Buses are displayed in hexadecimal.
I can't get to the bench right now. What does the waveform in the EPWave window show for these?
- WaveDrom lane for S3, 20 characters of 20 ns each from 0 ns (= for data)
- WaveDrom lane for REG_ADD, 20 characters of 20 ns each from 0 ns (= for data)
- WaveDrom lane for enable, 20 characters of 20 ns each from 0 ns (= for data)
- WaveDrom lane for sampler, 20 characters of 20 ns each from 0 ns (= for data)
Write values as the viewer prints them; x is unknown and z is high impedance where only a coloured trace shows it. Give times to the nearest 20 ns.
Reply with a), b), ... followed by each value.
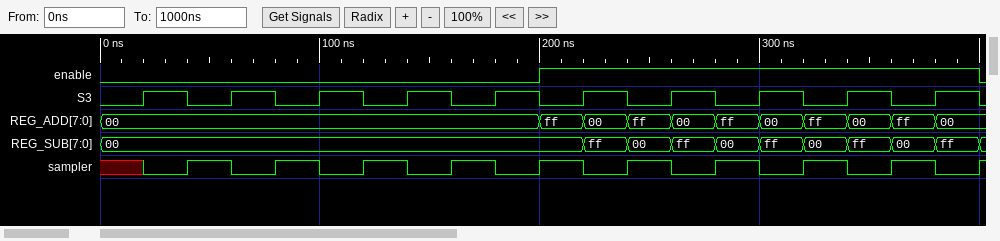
a) {name: 'S3', wave: '01010101010101010101'}
b) {name: 'REG_ADD', wave: '=.........==========', data: '00 ff 00 ff 00 ff 00 ff 00 ff 00'}
c) {name: 'enable', wave: '0.........1.........'}
d) {name: 'sampler', wave: 'x0101010101010101010'}
